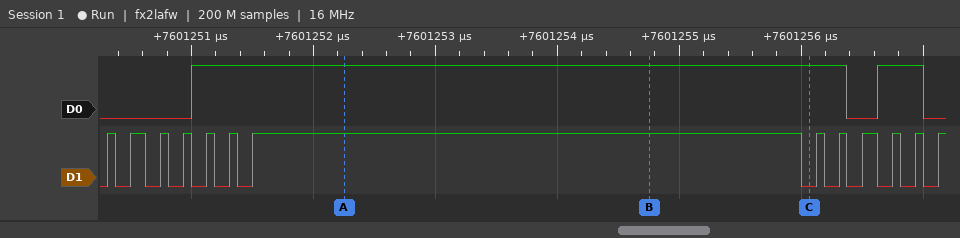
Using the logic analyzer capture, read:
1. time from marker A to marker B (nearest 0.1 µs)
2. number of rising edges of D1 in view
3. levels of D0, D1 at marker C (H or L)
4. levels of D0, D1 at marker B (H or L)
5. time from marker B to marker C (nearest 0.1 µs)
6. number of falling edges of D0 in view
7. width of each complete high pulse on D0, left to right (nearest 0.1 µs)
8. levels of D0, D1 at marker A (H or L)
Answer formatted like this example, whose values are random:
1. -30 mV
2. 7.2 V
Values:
1. 2.5 µs
2. 13
3. D0=H, D1=L
4. D0=H, D1=H
5. 1.3 µs
6. 2
7. 5.4 µs, 0.4 µs
8. D0=H, D1=H
